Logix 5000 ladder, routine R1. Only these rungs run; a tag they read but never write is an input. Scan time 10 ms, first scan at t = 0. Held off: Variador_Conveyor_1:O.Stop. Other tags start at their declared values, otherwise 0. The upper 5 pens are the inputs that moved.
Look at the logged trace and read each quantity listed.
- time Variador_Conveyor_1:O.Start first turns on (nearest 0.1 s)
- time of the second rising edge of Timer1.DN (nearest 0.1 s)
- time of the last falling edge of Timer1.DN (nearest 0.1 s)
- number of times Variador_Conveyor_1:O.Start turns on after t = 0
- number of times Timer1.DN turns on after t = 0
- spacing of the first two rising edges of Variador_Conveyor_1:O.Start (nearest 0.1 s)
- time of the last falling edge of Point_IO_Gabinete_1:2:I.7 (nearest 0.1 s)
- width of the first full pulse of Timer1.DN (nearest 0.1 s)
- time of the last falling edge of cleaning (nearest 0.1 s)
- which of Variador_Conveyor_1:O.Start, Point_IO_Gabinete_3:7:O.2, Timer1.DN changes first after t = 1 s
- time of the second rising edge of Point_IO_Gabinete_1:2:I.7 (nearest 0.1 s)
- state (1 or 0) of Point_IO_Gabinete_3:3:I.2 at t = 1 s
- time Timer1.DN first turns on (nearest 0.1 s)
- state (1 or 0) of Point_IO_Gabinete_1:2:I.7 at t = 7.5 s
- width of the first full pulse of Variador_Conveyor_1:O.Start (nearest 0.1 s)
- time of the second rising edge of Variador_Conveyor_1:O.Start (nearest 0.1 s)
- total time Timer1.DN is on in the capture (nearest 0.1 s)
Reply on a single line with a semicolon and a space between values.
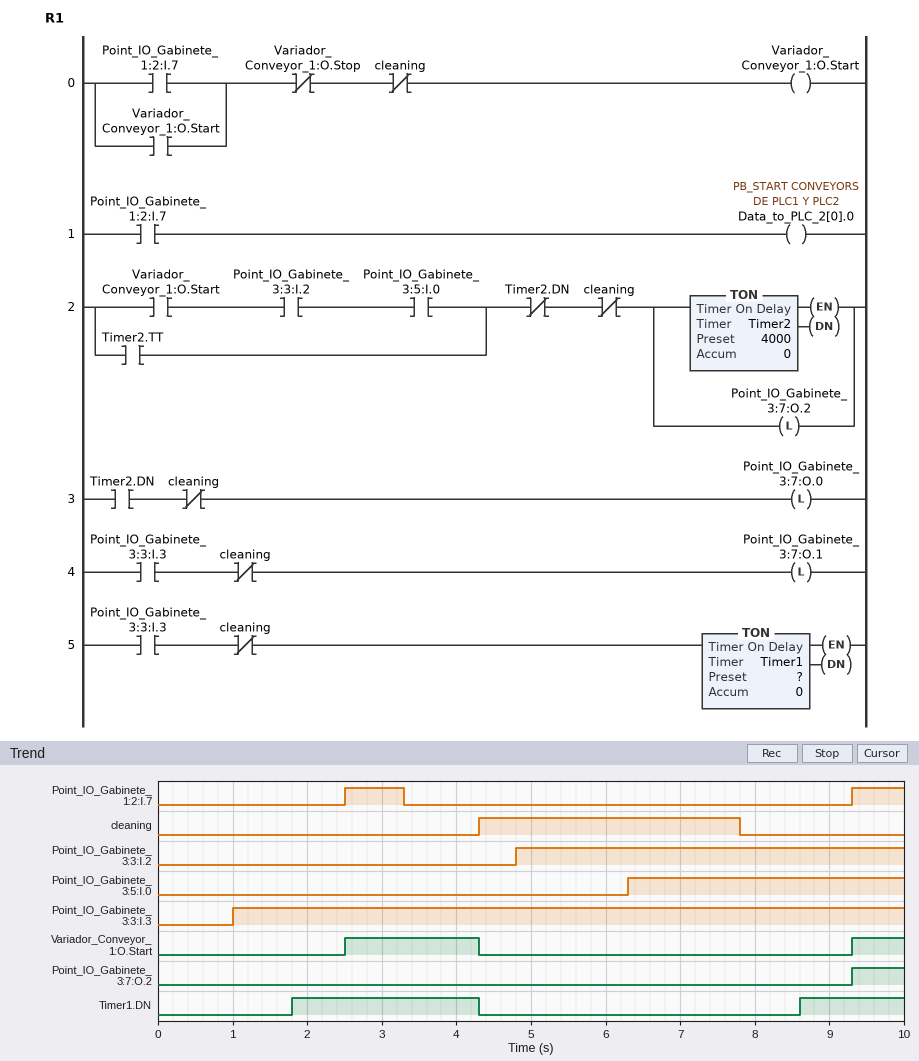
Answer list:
2.5 s; 8.6 s; 4.3 s; 2; 2; 6.8 s; 3.3 s; 2.5 s; 7.8 s; Timer1.DN; 9.3 s; 0; 1.8 s; 0; 1.8 s; 9.3 s; 3.9 s
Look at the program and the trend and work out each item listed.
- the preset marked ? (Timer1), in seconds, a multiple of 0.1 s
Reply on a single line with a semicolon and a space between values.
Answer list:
0.8 s
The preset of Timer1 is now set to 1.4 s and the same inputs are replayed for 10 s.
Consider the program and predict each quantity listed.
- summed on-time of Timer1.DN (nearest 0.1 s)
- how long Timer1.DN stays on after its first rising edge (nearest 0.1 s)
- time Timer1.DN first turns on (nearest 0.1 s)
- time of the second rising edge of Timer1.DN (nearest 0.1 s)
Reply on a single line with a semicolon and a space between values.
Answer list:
2.7 s; 1.9 s; 2.4 s; 9.2 s
